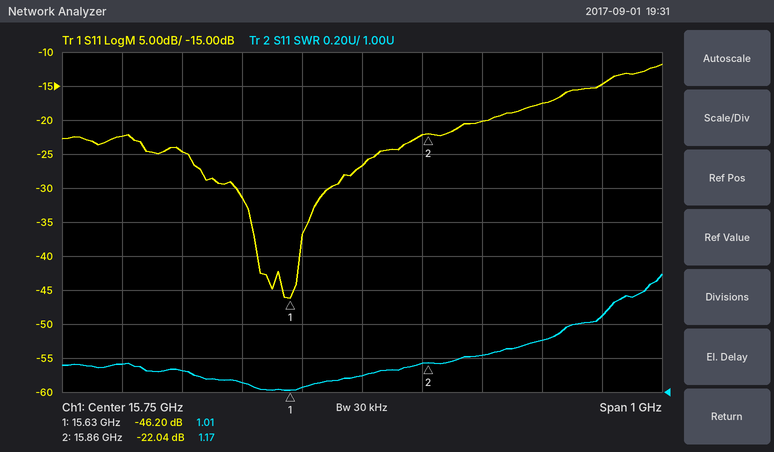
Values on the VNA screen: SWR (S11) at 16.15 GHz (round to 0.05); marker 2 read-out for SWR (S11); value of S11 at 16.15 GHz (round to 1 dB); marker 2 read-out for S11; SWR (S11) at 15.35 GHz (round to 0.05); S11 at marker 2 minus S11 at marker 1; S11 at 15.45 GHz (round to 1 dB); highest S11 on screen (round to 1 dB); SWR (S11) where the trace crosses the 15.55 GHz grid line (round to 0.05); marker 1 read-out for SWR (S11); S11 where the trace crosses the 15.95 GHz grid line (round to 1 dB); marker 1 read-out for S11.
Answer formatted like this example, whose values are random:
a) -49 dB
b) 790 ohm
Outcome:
a) 1.45
b) 1.17
c) -15 dB
d) -22.04 dB
e) 1.15
f) 24.16 dB
g) -25 dB
h) -12 dB
i) 1.05
j) 1.01
k) -20 dB
l) -46.20 dB
